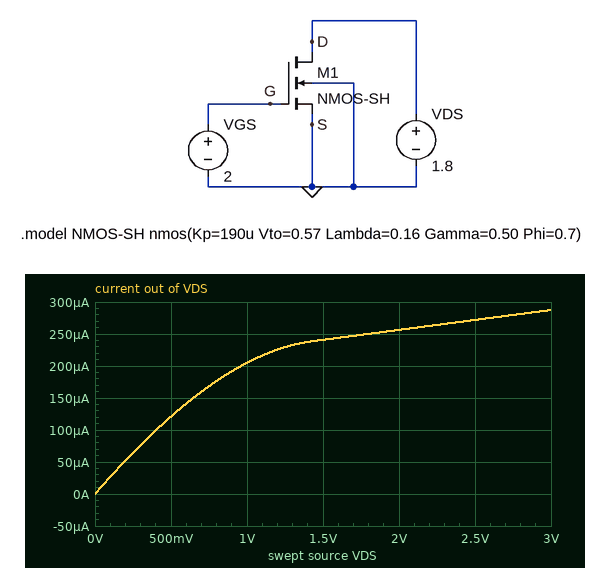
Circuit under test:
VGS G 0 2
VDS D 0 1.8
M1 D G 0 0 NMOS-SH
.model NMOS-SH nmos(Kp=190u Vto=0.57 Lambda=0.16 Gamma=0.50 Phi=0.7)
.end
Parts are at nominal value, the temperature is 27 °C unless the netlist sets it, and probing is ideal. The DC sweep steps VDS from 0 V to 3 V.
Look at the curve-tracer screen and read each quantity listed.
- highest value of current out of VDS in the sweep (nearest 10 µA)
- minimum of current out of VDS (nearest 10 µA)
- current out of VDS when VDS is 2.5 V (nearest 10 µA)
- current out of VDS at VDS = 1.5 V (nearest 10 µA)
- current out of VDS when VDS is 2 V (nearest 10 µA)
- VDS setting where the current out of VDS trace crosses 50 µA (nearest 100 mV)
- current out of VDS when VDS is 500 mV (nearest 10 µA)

290 µA
0 A
270 µA
240 µA
260 µA
200 mV
120 µA
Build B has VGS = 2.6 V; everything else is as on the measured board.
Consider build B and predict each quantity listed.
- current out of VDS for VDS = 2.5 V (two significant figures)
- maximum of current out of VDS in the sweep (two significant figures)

550 µA
580 µA
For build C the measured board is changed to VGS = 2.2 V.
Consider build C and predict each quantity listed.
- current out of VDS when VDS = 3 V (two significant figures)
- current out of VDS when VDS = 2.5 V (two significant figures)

370 µA
350 µA
